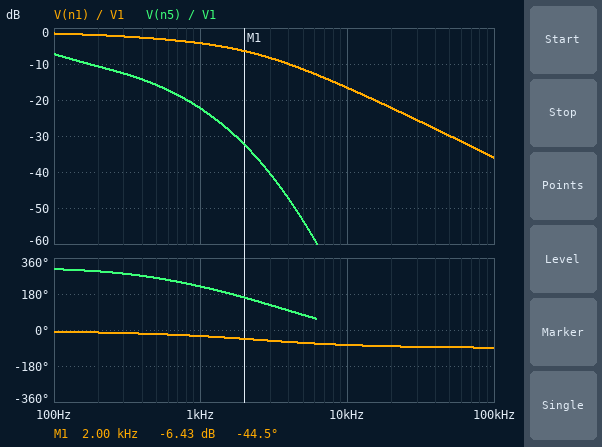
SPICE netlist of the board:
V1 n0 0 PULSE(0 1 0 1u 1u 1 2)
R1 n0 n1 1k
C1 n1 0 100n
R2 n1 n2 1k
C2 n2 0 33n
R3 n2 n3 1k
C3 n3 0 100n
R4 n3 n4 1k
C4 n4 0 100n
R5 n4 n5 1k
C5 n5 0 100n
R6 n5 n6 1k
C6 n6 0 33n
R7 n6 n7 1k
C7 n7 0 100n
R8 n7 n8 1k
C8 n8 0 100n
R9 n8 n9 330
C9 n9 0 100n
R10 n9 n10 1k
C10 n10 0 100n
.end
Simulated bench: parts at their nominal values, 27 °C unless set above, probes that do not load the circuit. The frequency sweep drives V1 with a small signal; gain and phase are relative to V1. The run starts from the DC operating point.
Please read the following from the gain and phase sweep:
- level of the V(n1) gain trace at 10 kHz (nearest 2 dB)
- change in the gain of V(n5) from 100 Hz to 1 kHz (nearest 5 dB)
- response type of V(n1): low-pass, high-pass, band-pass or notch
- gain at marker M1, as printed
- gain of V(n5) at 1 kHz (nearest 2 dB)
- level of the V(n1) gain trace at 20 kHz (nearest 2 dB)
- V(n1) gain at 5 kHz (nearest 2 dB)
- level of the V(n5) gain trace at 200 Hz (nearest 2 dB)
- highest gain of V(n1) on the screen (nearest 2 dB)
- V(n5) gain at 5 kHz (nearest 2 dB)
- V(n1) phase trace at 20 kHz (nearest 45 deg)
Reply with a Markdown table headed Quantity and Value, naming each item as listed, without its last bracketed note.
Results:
| Quantity | Value |
|---|---|
| level of the V(n1) gain trace at 10 kHz | -16 dB |
| change in the gain of V(n5) from 100 Hz to 1 kHz | -15 dB |
| response type of V(n1): low-pass, high-pass, band-pass or notch | low-pass |
| gain at marker M1, as printed | -6.43 dB |
| gain of V(n5) at 1 kHz | -22 dB |
| level of the V(n1) gain trace at 20 kHz | -22 dB |
| V(n1) gain at 5 kHz | -12 dB |
| level of the V(n5) gain trace at 200 Hz | -10 dB |
| highest gain of V(n1) on the screen | -2 dB |
| V(n5) gain at 5 kHz | -54 dB |
| V(n1) phase trace at 20 kHz | -90 deg |
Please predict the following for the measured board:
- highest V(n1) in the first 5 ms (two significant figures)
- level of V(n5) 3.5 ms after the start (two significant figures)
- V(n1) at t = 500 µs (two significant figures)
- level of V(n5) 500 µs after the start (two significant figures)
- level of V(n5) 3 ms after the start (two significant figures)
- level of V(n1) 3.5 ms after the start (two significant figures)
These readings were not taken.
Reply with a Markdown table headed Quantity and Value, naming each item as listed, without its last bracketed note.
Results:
| Quantity | Value |
|---|---|
| highest V(n1) in the first 5 ms | 950 mV |
| level of V(n5) 3.5 ms after the start | 640 mV |
| V(n1) at t = 500 µs | 780 mV |
| level of V(n5) 500 µs after the start | 150 mV |
| level of V(n5) 3 ms after the start | 600 mV |
| level of V(n1) 3.5 ms after the start | 920 mV |
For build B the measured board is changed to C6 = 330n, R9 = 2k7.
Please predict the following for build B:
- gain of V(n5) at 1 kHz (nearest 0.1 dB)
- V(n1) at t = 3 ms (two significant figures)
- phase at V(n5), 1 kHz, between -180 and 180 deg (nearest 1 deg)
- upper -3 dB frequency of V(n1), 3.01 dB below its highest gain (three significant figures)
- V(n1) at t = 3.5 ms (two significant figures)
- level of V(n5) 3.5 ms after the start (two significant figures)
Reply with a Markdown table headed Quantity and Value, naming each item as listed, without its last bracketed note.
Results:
| Quantity | Value |
|---|---|
| gain of V(n5) at 1 kHz | -24.3 dB |
| V(n1) at t = 3 ms | 890 mV |
| phase at V(n5), 1 kHz, between -180 and 180 deg | -135 deg |
| upper -3 dB frequency of V(n1), 3.01 dB below its highest gain | 528 Hz |
| V(n1) at t = 3.5 ms | 900 mV |
| level of V(n5) 3.5 ms after the start | 540 mV |
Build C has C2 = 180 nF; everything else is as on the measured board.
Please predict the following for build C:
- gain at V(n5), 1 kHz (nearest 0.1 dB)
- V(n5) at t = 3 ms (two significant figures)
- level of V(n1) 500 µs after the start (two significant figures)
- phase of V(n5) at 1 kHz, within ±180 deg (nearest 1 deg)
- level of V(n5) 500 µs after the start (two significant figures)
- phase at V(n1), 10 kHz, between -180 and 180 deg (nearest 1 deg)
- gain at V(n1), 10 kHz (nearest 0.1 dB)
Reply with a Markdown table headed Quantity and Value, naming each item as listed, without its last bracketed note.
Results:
| Quantity | Value |
|---|---|
| gain at V(n5), 1 kHz | -26.0 dB |
| V(n5) at t = 3 ms | 570 mV |
| level of V(n1) 500 µs after the start | 720 mV |
| phase of V(n5) at 1 kHz, within ±180 deg | -167 deg |
| level of V(n5) 500 µs after the start | 100 mV |
| phase at V(n1), 10 kHz, between -180 and 180 deg | -73 deg |
| gain at V(n1), 10 kHz | -16.5 dB |
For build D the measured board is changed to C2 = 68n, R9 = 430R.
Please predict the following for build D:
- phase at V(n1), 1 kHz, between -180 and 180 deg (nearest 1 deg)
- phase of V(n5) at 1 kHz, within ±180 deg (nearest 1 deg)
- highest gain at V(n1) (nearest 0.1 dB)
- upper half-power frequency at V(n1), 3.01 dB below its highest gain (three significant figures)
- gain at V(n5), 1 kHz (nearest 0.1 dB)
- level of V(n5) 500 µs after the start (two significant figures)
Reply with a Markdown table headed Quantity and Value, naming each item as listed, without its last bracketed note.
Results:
| Quantity | Value |
|---|---|
| phase at V(n1), 1 kHz, between -180 and 180 deg | -31 deg |
| phase of V(n5) at 1 kHz, within ±180 deg | -151 deg |
| highest gain at V(n1) | 0 dB |
| upper half-power frequency at V(n1), 3.01 dB below its highest gain | 429 Hz |
| gain at V(n5), 1 kHz | -23.2 dB |
| level of V(n5) 500 µs after the start | 140 mV |
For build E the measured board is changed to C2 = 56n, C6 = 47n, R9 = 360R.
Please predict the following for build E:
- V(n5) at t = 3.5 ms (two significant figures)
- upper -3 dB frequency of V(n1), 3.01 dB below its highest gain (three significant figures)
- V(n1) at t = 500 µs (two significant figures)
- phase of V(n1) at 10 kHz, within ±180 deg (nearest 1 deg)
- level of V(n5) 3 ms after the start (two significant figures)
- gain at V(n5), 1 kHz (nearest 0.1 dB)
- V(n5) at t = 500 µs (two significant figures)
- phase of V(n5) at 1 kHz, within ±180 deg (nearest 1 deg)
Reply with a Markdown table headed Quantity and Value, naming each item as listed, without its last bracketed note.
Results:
| Quantity | Value |
|---|---|
| V(n5) at t = 3.5 ms | 630 mV |
| upper -3 dB frequency of V(n1), 3.01 dB below its highest gain | 454 Hz |
| V(n1) at t = 500 µs | 770 mV |
| phase of V(n1) at 10 kHz, within ±180 deg | -74 deg |
| level of V(n5) 3 ms after the start | 590 mV |
| gain at V(n5), 1 kHz | -23.1 dB |
| V(n5) at t = 500 µs | 140 mV |
| phase of V(n5) at 1 kHz, within ±180 deg | -148 deg |
